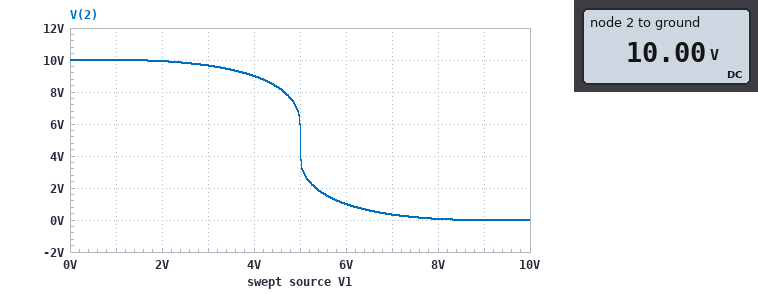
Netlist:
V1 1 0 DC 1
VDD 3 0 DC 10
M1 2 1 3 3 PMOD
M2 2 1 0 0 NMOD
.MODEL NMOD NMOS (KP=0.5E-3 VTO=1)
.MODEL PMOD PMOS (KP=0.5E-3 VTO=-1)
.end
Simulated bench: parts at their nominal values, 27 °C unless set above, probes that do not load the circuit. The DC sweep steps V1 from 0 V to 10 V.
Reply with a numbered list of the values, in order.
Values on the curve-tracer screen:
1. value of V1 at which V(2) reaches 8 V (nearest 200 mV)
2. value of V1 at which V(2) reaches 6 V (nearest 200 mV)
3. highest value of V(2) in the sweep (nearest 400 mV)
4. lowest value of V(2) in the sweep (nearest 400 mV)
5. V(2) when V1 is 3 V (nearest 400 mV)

1. 4.6 V
2. 5.0 V
3. 10.0 V
4. 0 V
5. 9.6 V
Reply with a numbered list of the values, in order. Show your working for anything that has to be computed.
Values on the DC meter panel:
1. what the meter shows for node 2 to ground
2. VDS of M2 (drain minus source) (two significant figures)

1. 10.00 V
2. 10 V = 10 V
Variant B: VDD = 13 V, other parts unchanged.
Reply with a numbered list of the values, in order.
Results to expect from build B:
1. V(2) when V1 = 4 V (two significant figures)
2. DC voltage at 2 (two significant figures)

1. 12 V
2. 13 V
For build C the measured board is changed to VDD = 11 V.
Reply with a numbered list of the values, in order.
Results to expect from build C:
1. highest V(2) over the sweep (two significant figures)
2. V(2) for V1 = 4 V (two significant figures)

1. 11 V
2. 10 V
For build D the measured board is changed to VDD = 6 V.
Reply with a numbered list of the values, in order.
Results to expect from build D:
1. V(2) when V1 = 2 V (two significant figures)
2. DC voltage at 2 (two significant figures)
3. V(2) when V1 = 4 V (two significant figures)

1. 5.8 V
2. 6.0 V
3. 170 mV
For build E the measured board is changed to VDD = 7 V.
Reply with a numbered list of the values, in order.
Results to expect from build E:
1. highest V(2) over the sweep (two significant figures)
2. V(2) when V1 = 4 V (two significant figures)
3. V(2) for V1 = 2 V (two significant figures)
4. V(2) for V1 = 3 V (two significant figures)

1. 7.0 V
2. 760 mV
3. 6.9 V
4. 6.2 V
